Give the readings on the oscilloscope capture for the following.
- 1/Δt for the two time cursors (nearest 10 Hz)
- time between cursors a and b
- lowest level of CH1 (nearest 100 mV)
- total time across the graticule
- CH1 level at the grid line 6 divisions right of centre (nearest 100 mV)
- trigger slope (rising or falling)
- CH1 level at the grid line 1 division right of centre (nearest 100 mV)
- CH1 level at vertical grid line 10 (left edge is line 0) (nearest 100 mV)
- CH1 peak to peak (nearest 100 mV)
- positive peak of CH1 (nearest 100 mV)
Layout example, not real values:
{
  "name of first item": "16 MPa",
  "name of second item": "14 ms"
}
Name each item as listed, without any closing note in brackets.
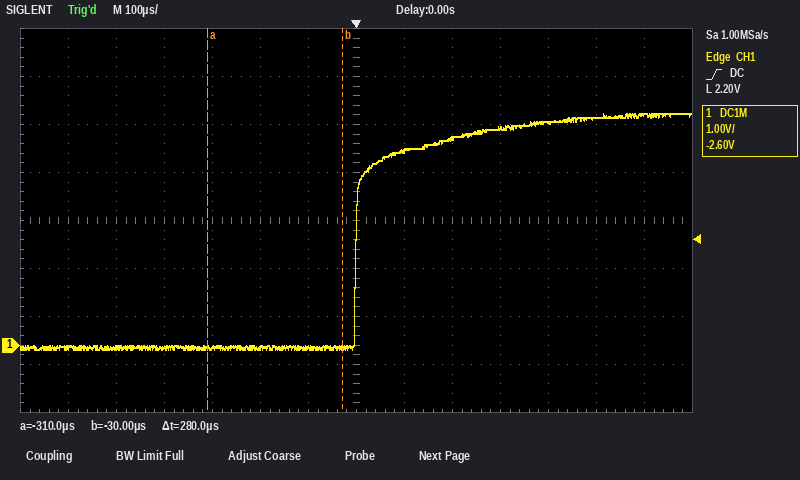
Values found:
{
  "1/Δt for the two time cursors": "3.57 kHz",
  "time between cursors a and b": "280 µs",
  "lowest level of CH1": "-100 mV",
  "total time across the graticule": "1.4 ms",
  "CH1 level at the grid line 6 divisions right of centre": "4.8 V",
  "trigger slope": "rising",
  "CH1 level at the grid line 1 division right of centre": "4.1 V",
  "CH1 level at vertical grid line 10 (left edge is line 0)": "4.5 V",
  "CH1 peak to peak": "4.9 V",
  "positive peak of CH1": "4.8 V"
}
